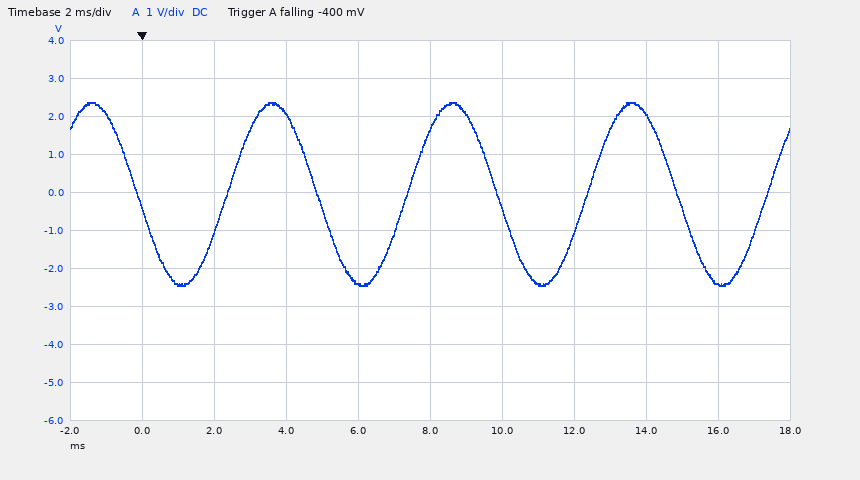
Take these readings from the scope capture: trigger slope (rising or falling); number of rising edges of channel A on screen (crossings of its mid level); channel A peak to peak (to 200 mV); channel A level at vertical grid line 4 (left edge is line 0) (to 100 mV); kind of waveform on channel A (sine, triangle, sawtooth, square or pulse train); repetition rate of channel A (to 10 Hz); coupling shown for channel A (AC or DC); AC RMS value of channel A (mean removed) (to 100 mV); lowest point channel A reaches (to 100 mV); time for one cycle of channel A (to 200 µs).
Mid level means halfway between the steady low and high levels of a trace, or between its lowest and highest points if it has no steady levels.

falling
4
4.8 V
-2.4 V
sine
200 Hz
DC
1.7 V
-2.4 V
5.0 ms
